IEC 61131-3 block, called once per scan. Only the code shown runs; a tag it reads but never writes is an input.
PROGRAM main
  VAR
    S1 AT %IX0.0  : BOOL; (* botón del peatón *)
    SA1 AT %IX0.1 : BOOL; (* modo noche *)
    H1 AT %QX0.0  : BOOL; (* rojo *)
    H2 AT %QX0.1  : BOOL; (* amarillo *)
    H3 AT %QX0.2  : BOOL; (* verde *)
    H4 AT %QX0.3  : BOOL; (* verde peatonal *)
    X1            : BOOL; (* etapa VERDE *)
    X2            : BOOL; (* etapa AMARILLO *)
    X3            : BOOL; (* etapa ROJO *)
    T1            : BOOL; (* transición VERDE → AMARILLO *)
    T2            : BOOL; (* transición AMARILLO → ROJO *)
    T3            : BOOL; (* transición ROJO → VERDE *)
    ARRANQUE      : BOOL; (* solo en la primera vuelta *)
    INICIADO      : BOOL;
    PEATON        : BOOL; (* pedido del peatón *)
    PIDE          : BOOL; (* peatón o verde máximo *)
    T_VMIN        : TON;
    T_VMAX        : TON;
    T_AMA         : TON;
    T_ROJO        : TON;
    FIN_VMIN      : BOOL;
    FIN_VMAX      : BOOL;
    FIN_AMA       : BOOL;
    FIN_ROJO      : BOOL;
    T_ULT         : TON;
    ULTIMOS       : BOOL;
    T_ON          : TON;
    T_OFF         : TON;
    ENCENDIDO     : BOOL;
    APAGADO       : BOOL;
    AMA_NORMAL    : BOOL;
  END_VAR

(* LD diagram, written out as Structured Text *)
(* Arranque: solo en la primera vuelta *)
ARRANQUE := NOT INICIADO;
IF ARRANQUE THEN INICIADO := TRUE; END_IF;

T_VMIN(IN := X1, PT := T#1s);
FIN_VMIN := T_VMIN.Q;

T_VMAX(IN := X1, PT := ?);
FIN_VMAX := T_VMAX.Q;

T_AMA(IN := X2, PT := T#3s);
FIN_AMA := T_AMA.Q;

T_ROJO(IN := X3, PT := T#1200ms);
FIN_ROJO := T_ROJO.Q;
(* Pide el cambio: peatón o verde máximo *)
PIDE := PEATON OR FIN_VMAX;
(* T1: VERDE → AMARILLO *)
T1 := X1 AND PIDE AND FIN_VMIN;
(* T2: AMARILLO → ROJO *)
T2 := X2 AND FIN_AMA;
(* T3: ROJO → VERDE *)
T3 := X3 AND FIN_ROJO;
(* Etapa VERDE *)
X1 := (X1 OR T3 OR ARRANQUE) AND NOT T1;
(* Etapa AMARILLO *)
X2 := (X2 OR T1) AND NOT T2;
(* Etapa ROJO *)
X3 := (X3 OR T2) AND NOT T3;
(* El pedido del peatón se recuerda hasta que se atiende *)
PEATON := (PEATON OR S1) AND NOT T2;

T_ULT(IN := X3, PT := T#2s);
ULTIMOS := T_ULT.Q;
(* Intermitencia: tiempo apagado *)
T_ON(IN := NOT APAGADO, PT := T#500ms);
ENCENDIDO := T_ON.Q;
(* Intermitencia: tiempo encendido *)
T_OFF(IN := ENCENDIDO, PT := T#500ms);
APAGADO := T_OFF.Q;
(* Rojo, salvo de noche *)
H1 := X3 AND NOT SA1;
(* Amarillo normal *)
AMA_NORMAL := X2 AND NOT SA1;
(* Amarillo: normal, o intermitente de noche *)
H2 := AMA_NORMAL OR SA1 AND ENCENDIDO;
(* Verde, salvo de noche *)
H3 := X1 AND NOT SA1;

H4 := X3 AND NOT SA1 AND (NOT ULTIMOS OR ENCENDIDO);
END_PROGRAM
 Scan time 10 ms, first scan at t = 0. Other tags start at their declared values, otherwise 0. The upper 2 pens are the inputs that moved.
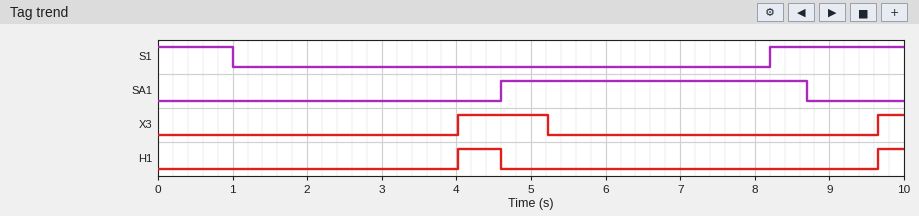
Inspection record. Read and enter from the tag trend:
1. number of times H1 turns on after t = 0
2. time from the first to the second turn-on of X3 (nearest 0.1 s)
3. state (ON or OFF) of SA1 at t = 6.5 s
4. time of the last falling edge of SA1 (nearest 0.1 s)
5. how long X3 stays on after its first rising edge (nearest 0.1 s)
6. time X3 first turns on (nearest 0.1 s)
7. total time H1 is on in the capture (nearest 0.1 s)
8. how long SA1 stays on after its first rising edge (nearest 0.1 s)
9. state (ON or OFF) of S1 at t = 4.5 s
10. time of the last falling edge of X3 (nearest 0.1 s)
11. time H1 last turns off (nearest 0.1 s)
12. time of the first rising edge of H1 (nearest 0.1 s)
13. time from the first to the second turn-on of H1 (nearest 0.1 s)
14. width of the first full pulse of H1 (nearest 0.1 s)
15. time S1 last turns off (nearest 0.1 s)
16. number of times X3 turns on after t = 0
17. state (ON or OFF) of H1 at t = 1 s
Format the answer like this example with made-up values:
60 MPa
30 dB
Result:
2
5.6 s
ON
8.7 s
1.2 s
4.0 s
0.9 s
4.1 s
OFF
5.2 s
4.6 s
4.0 s
5.6 s
0.6 s
1.0 s
2
OFF
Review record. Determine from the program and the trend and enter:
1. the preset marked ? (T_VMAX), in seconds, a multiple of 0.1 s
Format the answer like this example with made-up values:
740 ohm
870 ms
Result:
1.4 s
